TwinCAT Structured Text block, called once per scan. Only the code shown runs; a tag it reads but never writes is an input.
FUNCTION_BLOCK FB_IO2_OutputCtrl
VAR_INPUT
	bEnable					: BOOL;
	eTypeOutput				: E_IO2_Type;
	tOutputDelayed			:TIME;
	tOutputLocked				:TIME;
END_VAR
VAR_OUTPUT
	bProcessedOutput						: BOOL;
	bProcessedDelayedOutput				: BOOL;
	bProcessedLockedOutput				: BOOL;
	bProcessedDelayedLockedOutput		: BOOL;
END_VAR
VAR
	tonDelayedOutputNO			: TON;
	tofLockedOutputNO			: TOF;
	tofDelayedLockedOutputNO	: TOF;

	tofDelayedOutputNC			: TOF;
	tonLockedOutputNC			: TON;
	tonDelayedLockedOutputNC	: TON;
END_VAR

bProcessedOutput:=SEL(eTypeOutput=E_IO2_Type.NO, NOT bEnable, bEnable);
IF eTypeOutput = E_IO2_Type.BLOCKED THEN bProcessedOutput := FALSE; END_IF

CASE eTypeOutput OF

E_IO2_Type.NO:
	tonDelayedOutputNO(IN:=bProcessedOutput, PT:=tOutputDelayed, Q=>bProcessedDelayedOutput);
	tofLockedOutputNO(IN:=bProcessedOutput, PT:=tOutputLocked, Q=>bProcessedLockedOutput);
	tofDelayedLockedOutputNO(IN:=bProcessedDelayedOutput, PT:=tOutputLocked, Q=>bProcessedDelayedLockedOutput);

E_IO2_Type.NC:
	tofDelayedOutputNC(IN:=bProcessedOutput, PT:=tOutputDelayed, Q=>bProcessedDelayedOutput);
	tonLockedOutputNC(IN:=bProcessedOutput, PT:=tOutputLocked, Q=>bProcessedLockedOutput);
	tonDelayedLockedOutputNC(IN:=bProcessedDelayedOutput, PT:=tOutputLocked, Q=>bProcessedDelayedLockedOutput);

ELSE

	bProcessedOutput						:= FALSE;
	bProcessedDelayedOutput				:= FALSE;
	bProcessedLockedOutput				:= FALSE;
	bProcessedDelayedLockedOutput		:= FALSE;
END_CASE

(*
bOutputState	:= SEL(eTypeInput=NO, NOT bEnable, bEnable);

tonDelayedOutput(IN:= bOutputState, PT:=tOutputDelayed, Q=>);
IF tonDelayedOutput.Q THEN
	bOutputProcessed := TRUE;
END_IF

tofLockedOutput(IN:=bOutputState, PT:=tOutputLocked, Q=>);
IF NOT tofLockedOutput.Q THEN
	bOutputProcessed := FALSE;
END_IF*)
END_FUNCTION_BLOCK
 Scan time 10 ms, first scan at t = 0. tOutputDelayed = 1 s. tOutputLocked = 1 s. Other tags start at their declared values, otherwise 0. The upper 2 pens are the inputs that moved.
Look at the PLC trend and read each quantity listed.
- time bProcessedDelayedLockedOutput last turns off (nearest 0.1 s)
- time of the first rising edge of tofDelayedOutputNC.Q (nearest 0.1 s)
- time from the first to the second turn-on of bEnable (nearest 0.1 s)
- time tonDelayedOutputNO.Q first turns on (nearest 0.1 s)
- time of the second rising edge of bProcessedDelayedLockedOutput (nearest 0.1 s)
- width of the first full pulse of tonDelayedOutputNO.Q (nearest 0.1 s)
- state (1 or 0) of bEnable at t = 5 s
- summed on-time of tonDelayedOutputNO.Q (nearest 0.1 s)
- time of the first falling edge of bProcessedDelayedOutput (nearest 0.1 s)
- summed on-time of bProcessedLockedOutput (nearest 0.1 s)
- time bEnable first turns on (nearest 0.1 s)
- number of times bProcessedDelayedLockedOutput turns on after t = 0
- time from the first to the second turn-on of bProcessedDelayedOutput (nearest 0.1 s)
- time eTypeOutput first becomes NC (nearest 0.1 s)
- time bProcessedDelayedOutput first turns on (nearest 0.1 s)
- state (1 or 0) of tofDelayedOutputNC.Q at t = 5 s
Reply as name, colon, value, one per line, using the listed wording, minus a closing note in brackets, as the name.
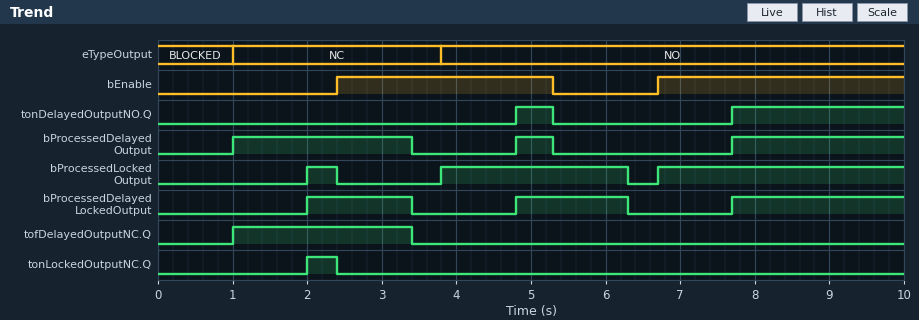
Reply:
time bProcessedDelayedLockedOutput last turns off: 6.3 s
time of the first rising edge of tofDelayedOutputNC.Q: 1.0 s
time from the first to the second turn-on of bEnable: 4.3 s
time tonDelayedOutputNO.Q first turns on: 4.8 s
time of the second rising edge of bProcessedDelayedLockedOutput: 4.8 s
width of the first full pulse of tonDelayedOutputNO.Q: 0.5 s
state (1 or 0) of bEnable at t = 5 s: 1
summed on-time of tonDelayedOutputNO.Q: 2.8 s
time of the first falling edge of bProcessedDelayedOutput: 3.4 s
summed on-time of bProcessedLockedOutput: 6.2 s
time bEnable first turns on: 2.4 s
number of times bProcessedDelayedLockedOutput turns on after t = 0: 3
time from the first to the second turn-on of bProcessedDelayedOutput: 3.8 s
time eTypeOutput first becomes NC: 1.0 s
time bProcessedDelayedOutput first turns on: 1.0 s
state (1 or 0) of tofDelayedOutputNC.Q at t = 5 s: 0
